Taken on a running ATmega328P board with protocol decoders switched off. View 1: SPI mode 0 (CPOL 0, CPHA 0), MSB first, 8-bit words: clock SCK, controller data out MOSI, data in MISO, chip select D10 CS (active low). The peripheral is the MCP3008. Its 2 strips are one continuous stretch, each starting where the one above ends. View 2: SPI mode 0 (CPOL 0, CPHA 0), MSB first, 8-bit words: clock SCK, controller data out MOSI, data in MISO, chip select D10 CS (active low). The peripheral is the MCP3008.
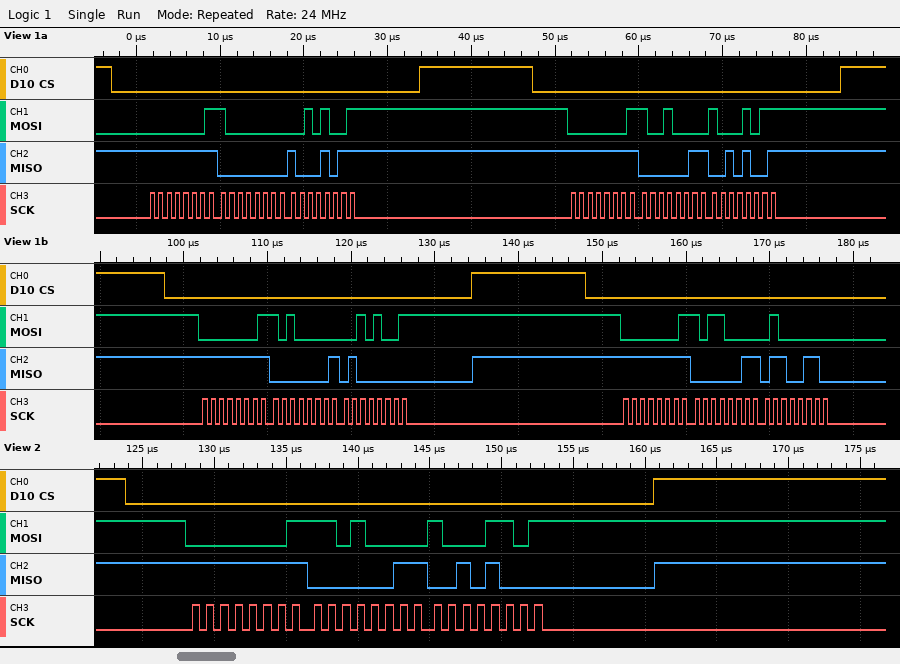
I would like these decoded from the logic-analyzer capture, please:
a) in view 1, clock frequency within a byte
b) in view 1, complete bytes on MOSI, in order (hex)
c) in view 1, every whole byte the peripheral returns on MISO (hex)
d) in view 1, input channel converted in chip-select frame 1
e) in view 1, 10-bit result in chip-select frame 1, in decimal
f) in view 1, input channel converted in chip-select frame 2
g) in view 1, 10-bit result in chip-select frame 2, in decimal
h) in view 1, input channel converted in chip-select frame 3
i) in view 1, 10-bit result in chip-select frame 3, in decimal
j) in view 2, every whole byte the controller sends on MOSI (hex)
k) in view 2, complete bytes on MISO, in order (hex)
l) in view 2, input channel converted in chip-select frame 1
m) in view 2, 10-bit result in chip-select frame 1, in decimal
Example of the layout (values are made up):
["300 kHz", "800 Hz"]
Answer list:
["1 MHz", "01 80 29 01 90 8B 01 A0 29 01 B0 40", "FF 00 8B FF 03 29 FF 01 40 FF 03 66", "0", "139", "1", "809", "2", "320", "0x01 0xD0 0x8D", "0xFF 0x03 0x28", "5", "808"]
